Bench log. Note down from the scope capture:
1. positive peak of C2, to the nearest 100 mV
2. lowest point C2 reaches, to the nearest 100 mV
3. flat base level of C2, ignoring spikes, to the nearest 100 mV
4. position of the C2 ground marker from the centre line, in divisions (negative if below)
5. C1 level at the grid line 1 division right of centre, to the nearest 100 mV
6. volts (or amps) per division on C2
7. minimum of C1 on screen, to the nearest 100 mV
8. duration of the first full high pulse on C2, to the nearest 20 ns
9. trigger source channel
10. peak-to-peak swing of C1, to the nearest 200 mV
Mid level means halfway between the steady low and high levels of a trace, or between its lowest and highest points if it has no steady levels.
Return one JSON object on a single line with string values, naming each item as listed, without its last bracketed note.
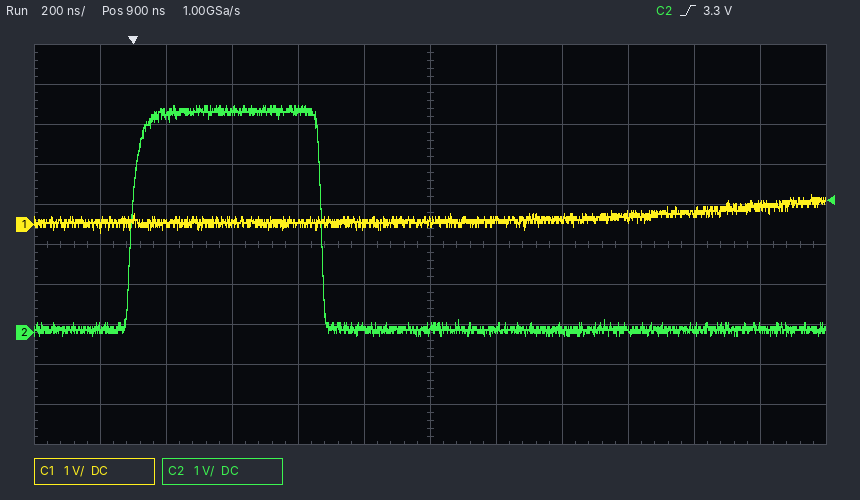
{"positive peak of C2, to the nearest 100 mV": "5.7 V", "lowest point C2 reaches, to the nearest 100 mV": "-100 mV", "flat base level of C2, ignoring spikes, to the nearest 100 mV": "100 mV", "position of the C2 ground marker from the centre line, in divisions": "-2.2 div", "C1 level at the grid line 1 division right of centre, to the nearest 100 mV": "100 mV", "volts (or amps) per division on C2": "1 V", "minimum of C1 on screen, to the nearest 100 mV": "-200 mV", "duration of the first full high pulse on C2, to the nearest 20 ns": "580 ns", "trigger source channel": "C2", "peak-to-peak swing of C1, to the nearest 200 mV": "1.0 V"}
